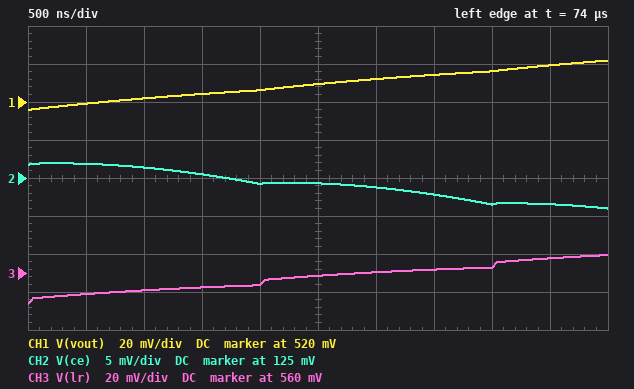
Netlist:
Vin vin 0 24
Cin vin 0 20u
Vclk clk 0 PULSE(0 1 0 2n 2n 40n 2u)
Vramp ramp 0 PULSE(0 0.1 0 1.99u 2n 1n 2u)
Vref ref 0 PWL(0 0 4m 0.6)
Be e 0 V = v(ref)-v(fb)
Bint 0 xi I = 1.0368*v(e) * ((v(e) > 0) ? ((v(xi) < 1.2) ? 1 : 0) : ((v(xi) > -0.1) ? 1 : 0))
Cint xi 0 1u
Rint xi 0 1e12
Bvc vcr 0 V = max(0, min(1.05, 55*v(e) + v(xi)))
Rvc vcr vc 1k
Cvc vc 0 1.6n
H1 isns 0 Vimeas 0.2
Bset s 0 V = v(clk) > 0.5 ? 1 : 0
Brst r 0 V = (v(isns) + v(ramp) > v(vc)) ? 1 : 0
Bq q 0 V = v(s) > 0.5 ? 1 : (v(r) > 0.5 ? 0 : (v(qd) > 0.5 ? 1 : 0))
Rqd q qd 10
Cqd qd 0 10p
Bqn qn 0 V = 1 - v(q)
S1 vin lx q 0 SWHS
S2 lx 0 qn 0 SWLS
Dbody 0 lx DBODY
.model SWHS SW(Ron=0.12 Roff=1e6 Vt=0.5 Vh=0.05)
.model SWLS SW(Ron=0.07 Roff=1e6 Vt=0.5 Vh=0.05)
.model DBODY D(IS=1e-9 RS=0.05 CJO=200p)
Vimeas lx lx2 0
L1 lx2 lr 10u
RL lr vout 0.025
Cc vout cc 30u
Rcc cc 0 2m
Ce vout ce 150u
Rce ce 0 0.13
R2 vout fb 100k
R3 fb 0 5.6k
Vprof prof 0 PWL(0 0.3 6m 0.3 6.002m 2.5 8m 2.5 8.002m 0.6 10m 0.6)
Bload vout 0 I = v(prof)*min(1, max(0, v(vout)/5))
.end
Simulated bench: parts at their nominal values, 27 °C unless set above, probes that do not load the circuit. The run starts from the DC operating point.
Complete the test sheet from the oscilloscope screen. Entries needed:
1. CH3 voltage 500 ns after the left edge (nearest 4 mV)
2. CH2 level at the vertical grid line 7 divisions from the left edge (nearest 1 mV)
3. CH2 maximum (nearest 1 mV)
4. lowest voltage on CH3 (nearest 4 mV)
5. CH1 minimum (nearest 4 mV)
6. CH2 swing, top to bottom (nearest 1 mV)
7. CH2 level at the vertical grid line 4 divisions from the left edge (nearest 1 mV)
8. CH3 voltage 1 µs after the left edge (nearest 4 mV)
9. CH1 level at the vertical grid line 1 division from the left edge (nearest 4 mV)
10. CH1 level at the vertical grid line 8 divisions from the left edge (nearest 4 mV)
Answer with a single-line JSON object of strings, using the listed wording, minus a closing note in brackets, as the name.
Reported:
{"CH3 voltage 500 ns after the left edge": "548 mV", "CH2 level at the vertical grid line 7 divisions from the left edge": "123 mV", "CH2 maximum": "127 mV", "lowest voltage on CH3": "544 mV", "CH1 minimum": "516 mV", "CH2 swing, top to bottom": "6 mV", "CH2 level at the vertical grid line 4 divisions from the left edge": "124 mV", "CH3 voltage 1 µs after the left edge": "552 mV", "CH1 level at the vertical grid line 1 division from the left edge": "520 mV", "CH1 level at the vertical grid line 8 divisions from the left edge": "536 mV"}
